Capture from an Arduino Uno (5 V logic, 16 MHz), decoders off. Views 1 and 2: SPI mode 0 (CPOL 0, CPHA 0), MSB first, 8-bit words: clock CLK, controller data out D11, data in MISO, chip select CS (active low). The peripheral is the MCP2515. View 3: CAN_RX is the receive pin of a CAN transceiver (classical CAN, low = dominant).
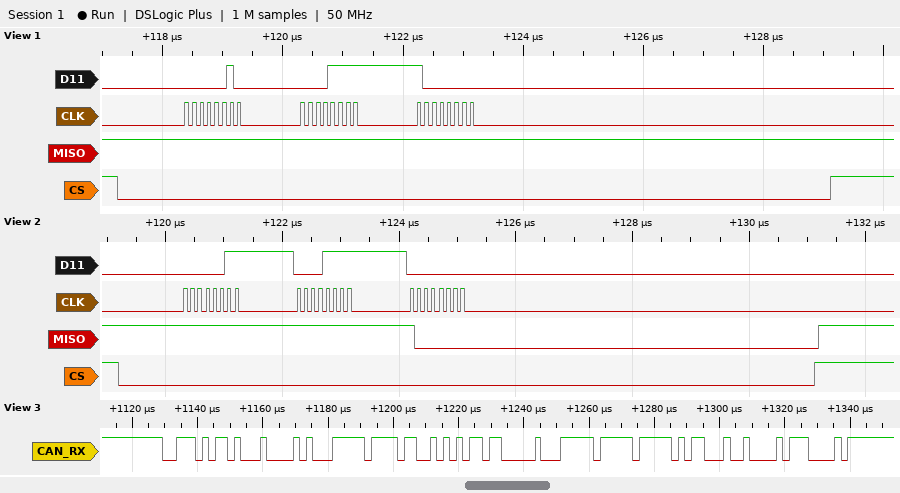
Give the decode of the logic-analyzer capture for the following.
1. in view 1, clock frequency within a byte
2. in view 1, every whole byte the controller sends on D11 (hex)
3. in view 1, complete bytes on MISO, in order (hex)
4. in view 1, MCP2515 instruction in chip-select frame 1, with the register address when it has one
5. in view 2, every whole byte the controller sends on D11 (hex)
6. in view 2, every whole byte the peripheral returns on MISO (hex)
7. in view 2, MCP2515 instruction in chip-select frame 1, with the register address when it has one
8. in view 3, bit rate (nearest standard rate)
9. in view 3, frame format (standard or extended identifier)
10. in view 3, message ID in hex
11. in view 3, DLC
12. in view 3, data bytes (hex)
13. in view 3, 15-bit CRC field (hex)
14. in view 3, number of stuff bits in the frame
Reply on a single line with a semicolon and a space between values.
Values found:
8 MHz; 0x02 0x0F 0x80; 0xFF 0xFF 0xFF; WRITE 0x0F; 03 0F 00; FF FF 80; READ 0x0F; 500 kbit/s; standard; 0x3AD; 8; 51 FF 65 5B 00 FF FF 62; 0x2170; 5
